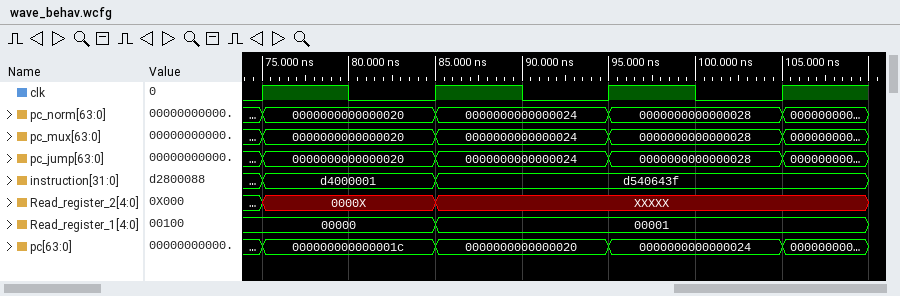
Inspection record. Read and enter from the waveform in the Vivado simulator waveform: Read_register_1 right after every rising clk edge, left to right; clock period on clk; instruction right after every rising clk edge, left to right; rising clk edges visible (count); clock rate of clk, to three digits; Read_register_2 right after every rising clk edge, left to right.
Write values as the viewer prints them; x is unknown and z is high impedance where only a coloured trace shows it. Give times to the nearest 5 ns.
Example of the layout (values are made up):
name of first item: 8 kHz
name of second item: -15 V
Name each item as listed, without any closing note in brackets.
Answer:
Read_register_1 right after every rising clk edge, left to right: 00000, 00001, 00001, 00001
clock period on clk: 10 ns
instruction right after every rising clk edge, left to right: d4000001, d540643f, d540643f, d540643f
rising clk edges visible: 4
clock rate of clk, to three digits: 100 MHz
Read_register_2 right after every rising clk edge, left to right: 0000X, XXXXX, XXXXX, XXXXX
